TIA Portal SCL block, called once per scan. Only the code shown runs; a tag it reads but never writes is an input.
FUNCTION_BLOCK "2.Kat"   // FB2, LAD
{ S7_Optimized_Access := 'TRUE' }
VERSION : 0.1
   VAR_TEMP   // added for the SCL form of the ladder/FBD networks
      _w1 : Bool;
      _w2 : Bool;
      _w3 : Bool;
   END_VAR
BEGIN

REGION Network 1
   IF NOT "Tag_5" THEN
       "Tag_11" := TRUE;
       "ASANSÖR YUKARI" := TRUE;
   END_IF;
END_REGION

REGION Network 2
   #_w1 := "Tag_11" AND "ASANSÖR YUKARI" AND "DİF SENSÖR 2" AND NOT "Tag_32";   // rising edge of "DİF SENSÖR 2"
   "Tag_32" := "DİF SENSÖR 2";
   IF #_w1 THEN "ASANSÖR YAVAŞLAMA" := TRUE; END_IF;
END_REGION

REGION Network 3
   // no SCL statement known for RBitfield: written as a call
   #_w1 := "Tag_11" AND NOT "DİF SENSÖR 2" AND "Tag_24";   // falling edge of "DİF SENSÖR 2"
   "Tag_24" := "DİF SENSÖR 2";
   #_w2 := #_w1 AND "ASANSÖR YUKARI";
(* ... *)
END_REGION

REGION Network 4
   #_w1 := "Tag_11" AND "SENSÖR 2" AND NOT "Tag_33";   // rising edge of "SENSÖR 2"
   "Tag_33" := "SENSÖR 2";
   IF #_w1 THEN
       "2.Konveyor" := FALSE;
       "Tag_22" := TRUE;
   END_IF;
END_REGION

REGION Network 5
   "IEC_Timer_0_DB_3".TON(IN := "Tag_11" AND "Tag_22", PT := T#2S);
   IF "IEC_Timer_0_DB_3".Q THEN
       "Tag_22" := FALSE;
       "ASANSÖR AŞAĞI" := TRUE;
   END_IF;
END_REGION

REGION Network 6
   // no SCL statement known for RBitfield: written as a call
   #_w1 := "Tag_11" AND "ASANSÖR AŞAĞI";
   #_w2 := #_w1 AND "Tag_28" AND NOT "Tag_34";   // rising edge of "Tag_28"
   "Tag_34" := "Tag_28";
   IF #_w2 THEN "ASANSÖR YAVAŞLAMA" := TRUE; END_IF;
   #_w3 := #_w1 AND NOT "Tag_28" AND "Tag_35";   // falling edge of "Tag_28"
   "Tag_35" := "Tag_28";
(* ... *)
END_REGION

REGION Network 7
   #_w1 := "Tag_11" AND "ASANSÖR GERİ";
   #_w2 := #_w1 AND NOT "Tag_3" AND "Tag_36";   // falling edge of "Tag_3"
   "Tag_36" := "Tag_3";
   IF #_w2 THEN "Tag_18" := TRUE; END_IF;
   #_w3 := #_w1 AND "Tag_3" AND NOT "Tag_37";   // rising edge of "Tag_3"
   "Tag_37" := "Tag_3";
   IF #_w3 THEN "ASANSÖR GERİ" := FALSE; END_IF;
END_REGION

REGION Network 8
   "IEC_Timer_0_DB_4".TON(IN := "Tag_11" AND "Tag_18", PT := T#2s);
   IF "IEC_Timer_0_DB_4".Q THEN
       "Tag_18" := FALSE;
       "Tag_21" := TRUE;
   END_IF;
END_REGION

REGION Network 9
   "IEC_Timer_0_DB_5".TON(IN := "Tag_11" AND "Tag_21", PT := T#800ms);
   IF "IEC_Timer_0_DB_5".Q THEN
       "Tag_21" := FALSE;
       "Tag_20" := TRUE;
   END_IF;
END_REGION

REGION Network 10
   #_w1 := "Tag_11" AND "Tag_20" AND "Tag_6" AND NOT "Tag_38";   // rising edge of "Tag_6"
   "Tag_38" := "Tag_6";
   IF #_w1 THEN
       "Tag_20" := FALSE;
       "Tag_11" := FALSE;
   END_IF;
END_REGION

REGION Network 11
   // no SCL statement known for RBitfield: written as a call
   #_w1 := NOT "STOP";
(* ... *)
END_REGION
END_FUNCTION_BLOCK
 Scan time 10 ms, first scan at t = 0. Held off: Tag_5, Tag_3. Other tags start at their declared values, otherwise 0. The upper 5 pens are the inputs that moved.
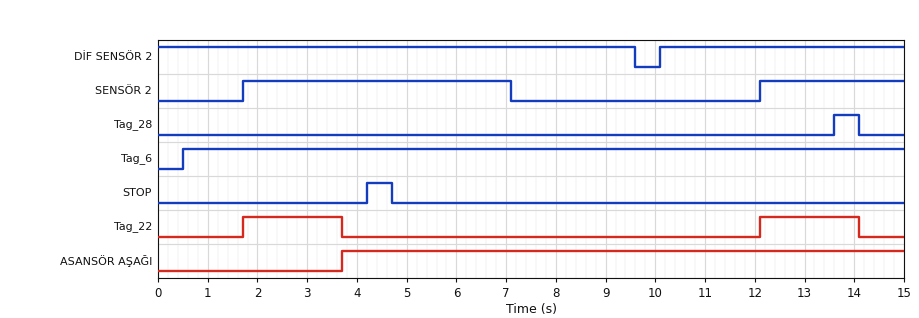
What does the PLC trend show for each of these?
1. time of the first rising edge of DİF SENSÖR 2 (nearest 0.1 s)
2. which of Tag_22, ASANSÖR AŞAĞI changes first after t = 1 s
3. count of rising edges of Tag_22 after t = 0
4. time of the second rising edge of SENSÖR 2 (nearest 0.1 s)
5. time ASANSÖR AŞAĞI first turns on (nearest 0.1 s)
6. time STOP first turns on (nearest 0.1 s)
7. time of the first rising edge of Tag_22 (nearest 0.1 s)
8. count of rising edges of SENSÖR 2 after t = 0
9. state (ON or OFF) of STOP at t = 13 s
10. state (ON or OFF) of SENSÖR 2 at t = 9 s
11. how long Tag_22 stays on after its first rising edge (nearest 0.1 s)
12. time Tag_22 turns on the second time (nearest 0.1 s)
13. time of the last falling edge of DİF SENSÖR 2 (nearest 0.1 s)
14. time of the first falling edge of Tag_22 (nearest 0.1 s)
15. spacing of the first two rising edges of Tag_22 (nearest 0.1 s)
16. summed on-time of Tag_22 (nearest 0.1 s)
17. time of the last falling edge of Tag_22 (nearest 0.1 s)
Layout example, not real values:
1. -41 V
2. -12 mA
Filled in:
1. 10.1 s
2. Tag_22
3. 2
4. 12.1 s
5. 3.7 s
6. 4.2 s
7. 1.7 s
8. 2
9. OFF
10. OFF
11. 2.0 s
12. 12.1 s
13. 9.6 s
14. 3.7 s
15. 10.4 s
16. 4.0 s
17. 14.1 s
